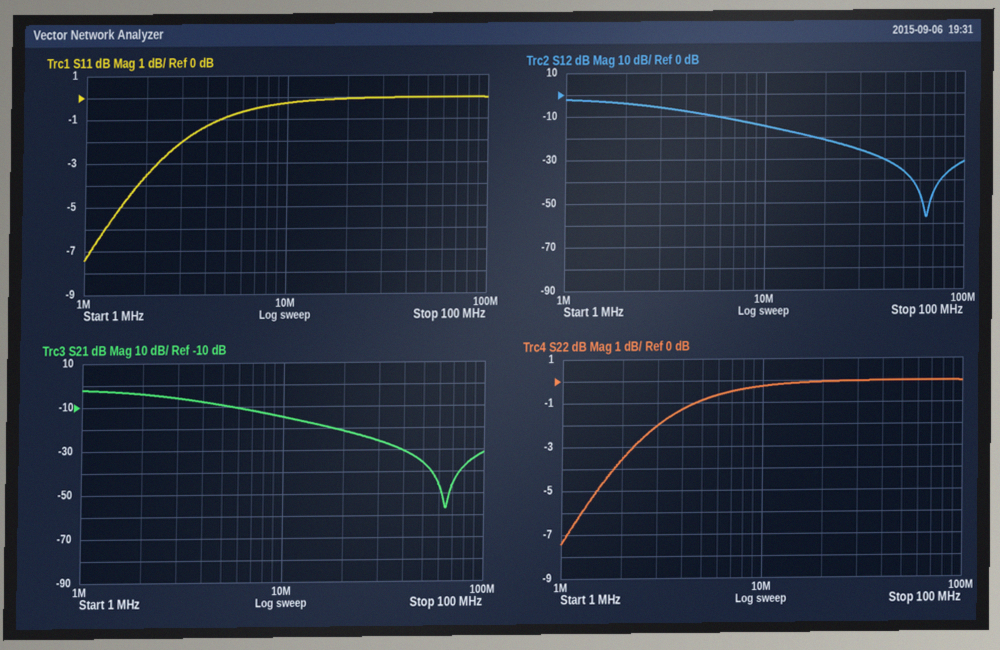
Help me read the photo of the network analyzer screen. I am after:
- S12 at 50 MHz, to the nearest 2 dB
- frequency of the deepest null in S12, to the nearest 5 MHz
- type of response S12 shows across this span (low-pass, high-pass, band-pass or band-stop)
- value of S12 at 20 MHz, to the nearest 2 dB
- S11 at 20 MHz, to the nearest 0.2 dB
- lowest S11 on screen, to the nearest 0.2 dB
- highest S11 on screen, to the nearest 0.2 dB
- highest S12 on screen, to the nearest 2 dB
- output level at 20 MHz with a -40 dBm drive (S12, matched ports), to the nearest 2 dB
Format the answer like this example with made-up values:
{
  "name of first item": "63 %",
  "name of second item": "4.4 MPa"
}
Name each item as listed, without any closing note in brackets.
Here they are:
{
  "S12 at 50 MHz, to the nearest 2 dB": "-36 dB",
  "frequency of the deepest null in S12, to the nearest 5 MHz": "65 MHz",
  "type of response S12 shows across this span": "low-pass",
  "value of S12 at 20 MHz, to the nearest 2 dB": "-22 dB",
  "S11 at 20 MHz, to the nearest 0.2 dB": "0.0 dB",
  "lowest S11 on screen, to the nearest 0.2 dB": "-7.4 dB",
  "highest S11 on screen, to the nearest 0.2 dB": "0.0 dB",
  "highest S12 on screen, to the nearest 2 dB": "-2 dB",
  "output level at 20 MHz with a -40 dBm drive (S12, matched ports), to the nearest 2 dB": "-62 dBm"
}
